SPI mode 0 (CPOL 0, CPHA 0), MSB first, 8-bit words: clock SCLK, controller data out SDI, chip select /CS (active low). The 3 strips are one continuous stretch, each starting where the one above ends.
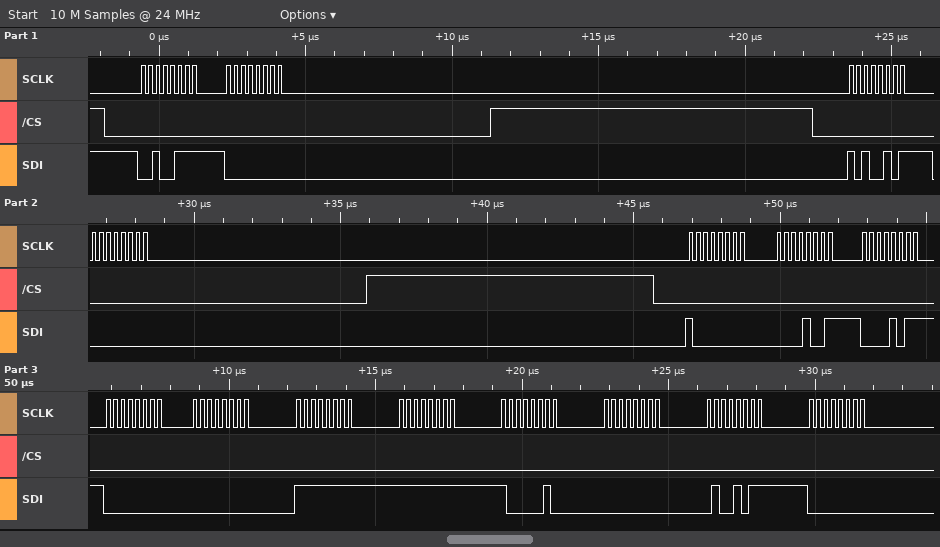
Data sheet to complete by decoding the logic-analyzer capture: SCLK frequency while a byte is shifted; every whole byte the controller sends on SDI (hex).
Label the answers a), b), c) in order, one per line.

a) 4 MHz
b) 27 00 A5 00 80 09 0B 00 00 FF FF 82 00 4B 00
